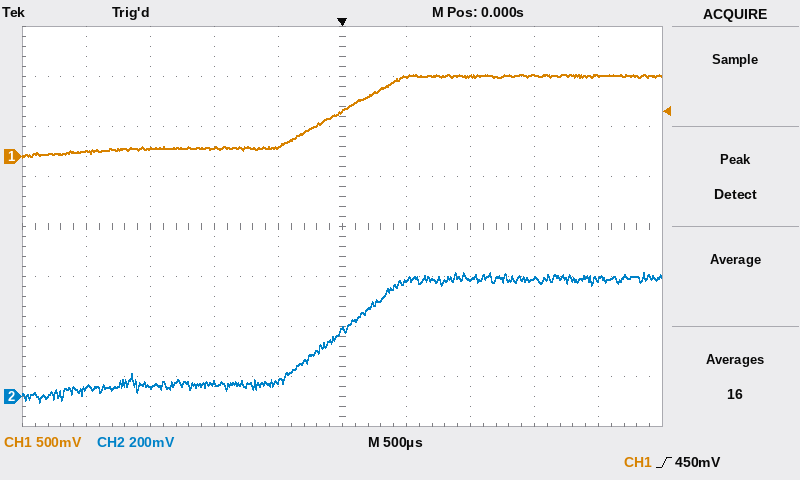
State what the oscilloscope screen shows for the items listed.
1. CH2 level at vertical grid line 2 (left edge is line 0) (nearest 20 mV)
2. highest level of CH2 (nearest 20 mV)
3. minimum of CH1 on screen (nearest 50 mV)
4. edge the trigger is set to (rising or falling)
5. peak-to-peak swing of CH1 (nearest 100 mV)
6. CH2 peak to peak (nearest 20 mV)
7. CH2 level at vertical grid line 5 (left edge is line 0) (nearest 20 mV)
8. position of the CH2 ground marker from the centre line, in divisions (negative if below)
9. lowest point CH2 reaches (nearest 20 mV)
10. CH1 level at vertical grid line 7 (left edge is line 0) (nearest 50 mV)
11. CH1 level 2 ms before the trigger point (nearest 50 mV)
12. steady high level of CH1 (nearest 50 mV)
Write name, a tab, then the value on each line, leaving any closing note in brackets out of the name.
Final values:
CH2 level at vertical grid line 2 (left edge is line 0)	40 mV
highest level of CH2	500 mV
minimum of CH1 on screen	0 mV
edge the trigger is set to	rising
peak-to-peak swing of CH1	800 mV
CH2 peak to peak	520 mV
CH2 level at vertical grid line 5 (left edge is line 0)	260 mV
position of the CH2 ground marker from the centre line, in divisions	-3.4 div
lowest point CH2 reaches	-20 mV
CH1 level at vertical grid line 7 (left edge is line 0)	800 mV
CH1 level 2 ms before the trigger point	50 mV
steady high level of CH1	800 mV
